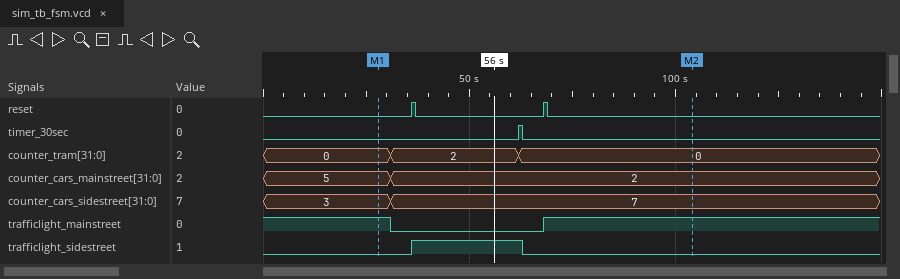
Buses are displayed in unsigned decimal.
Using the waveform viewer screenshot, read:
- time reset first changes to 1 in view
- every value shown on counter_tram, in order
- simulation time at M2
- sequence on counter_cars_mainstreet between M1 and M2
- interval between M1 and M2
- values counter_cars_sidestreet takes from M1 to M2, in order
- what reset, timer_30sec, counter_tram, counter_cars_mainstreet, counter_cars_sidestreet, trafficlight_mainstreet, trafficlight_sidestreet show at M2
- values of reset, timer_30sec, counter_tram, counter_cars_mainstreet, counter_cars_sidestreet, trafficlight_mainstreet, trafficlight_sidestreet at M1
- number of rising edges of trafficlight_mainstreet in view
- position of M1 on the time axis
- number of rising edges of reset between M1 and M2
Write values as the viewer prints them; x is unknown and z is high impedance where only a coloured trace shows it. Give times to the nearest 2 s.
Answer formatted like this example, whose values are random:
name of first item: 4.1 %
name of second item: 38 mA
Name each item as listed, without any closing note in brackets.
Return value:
time reset first changes to 1 in view: 36 s
every value shown on counter_tram, in order: 0, 2, 0
simulation time at M2: 104 s
sequence on counter_cars_mainstreet between M1 and M2: 5, 2
interval between M1 and M2: 76 s
values counter_cars_sidestreet takes from M1 to M2, in order: 3, 7
what reset, timer_30sec, counter_tram, counter_cars_mainstreet, counter_cars_sidestreet, trafficlight_mainstreet, trafficlight_sidestreet show at M2: reset=0, timer_30sec=0, counter_tram=0, counter_cars_mainstreet=2, counter_cars_sidestreet=7, trafficlight_mainstreet=1, trafficlight_sidestreet=0
values of reset, timer_30sec, counter_tram, counter_cars_mainstreet, counter_cars_sidestreet, trafficlight_mainstreet, trafficlight_sidestreet at M1: reset=0, timer_30sec=0, counter_tram=0, counter_cars_mainstreet=5, counter_cars_sidestreet=3, trafficlight_mainstreet=1, trafficlight_sidestreet=0
number of rising edges of trafficlight_mainstreet in view: 1
position of M1 on the time axis: 28 s
number of rising edges of reset between M1 and M2: 2
